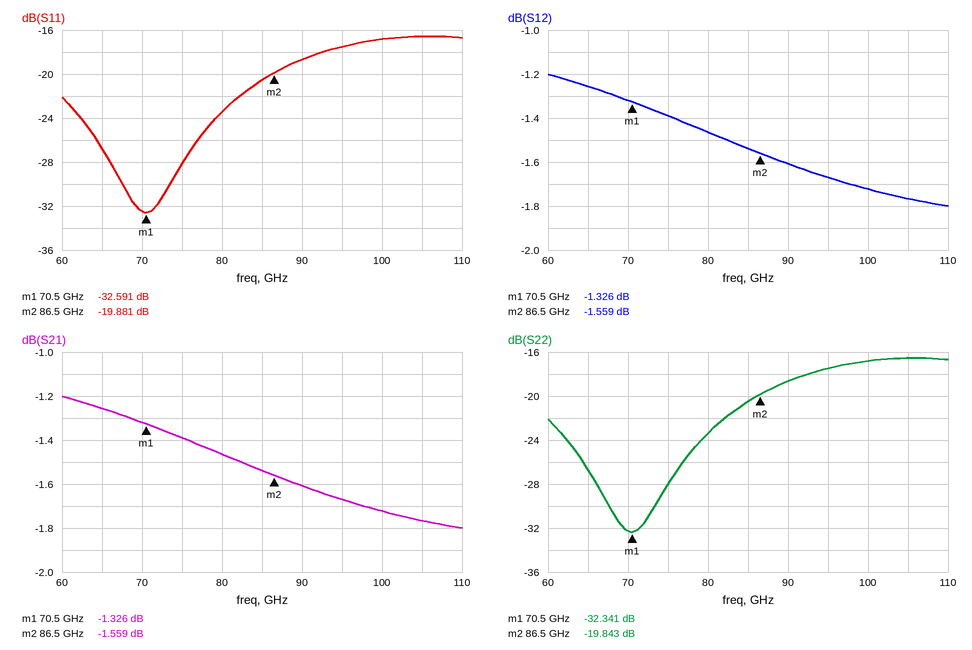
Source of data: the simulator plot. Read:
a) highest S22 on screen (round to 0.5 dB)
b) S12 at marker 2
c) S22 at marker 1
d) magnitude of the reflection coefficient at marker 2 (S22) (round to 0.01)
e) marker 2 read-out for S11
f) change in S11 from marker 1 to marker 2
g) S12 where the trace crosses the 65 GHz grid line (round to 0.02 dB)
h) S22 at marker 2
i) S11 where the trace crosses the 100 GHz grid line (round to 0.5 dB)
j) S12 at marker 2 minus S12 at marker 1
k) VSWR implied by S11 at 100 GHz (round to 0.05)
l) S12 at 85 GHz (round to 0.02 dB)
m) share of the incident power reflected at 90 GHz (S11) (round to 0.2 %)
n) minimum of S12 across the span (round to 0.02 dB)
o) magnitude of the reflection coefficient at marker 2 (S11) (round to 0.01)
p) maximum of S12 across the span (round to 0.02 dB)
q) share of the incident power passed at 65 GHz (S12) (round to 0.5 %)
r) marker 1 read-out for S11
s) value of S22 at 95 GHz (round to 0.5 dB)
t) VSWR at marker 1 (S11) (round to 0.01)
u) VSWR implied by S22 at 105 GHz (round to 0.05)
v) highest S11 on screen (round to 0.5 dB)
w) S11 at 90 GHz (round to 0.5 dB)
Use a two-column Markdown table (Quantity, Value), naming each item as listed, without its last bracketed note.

| Quantity | Value |
|---|---|
| highest S22 on screen | -16.5 dB |
| S12 at marker 2 | -1.559 dB |
| S22 at marker 1 | -32.341 dB |
| magnitude of the reflection coefficient at marker 2 (S22) | 0.10 |
| marker 2 read-out for S11 | -19.881 dB |
| change in S11 from marker 1 to marker 2 | 12.710 dB |
| S12 where the trace crosses the 65 GHz grid line | -1.26 dB |
| S22 at marker 2 | -19.843 dB |
| S11 where the trace crosses the 100 GHz grid line | -17.0 dB |
| S12 at marker 2 minus S12 at marker 1 | -0.233 dB |
| VSWR implied by S11 at 100 GHz | 1.35 |
| S12 at 85 GHz | -1.54 dB |
| share of the incident power reflected at 90 GHz (S11) | 1.4 % |
| minimum of S12 across the span | -1.80 dB |
| magnitude of the reflection coefficient at marker 2 (S11) | 0.10 |
| maximum of S12 across the span | -1.20 dB |
| share of the incident power passed at 65 GHz (S12) | 75.0 % |
| marker 1 read-out for S11 | -32.591 dB |
| value of S22 at 95 GHz | -17.5 dB |
| VSWR at marker 1 (S11) | 1.05 |
| VSWR implied by S22 at 105 GHz | 1.35 |
| highest S11 on screen | -16.5 dB |
| S11 at 90 GHz | -18.5 dB |
